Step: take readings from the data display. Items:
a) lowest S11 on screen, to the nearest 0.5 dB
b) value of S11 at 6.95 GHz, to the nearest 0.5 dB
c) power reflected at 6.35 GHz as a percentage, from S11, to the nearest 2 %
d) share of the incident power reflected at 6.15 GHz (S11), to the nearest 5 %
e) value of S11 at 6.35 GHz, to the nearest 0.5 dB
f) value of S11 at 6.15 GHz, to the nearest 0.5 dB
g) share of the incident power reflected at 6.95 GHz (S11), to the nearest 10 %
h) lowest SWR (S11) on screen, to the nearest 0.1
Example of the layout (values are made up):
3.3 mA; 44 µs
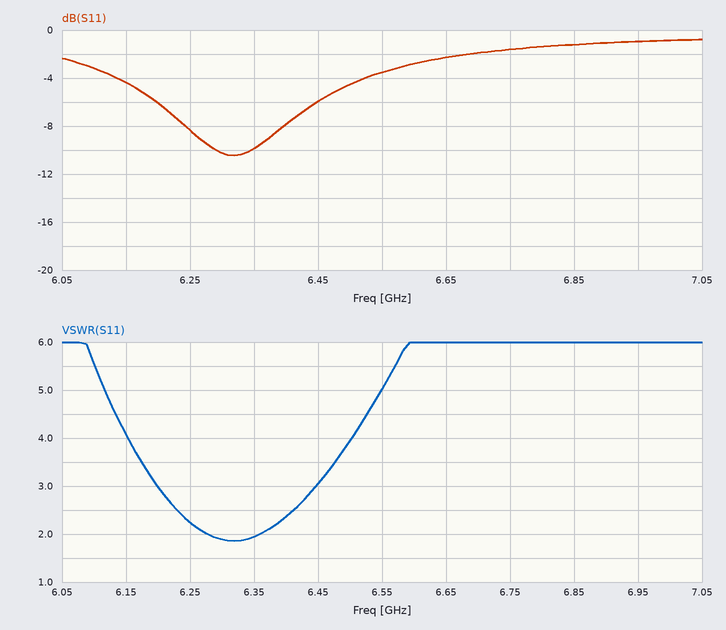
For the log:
-10.5 dB; -1.0 dB; 10 %; 35 %; -10.0 dB; -4.5 dB; 80 %; 1.9
